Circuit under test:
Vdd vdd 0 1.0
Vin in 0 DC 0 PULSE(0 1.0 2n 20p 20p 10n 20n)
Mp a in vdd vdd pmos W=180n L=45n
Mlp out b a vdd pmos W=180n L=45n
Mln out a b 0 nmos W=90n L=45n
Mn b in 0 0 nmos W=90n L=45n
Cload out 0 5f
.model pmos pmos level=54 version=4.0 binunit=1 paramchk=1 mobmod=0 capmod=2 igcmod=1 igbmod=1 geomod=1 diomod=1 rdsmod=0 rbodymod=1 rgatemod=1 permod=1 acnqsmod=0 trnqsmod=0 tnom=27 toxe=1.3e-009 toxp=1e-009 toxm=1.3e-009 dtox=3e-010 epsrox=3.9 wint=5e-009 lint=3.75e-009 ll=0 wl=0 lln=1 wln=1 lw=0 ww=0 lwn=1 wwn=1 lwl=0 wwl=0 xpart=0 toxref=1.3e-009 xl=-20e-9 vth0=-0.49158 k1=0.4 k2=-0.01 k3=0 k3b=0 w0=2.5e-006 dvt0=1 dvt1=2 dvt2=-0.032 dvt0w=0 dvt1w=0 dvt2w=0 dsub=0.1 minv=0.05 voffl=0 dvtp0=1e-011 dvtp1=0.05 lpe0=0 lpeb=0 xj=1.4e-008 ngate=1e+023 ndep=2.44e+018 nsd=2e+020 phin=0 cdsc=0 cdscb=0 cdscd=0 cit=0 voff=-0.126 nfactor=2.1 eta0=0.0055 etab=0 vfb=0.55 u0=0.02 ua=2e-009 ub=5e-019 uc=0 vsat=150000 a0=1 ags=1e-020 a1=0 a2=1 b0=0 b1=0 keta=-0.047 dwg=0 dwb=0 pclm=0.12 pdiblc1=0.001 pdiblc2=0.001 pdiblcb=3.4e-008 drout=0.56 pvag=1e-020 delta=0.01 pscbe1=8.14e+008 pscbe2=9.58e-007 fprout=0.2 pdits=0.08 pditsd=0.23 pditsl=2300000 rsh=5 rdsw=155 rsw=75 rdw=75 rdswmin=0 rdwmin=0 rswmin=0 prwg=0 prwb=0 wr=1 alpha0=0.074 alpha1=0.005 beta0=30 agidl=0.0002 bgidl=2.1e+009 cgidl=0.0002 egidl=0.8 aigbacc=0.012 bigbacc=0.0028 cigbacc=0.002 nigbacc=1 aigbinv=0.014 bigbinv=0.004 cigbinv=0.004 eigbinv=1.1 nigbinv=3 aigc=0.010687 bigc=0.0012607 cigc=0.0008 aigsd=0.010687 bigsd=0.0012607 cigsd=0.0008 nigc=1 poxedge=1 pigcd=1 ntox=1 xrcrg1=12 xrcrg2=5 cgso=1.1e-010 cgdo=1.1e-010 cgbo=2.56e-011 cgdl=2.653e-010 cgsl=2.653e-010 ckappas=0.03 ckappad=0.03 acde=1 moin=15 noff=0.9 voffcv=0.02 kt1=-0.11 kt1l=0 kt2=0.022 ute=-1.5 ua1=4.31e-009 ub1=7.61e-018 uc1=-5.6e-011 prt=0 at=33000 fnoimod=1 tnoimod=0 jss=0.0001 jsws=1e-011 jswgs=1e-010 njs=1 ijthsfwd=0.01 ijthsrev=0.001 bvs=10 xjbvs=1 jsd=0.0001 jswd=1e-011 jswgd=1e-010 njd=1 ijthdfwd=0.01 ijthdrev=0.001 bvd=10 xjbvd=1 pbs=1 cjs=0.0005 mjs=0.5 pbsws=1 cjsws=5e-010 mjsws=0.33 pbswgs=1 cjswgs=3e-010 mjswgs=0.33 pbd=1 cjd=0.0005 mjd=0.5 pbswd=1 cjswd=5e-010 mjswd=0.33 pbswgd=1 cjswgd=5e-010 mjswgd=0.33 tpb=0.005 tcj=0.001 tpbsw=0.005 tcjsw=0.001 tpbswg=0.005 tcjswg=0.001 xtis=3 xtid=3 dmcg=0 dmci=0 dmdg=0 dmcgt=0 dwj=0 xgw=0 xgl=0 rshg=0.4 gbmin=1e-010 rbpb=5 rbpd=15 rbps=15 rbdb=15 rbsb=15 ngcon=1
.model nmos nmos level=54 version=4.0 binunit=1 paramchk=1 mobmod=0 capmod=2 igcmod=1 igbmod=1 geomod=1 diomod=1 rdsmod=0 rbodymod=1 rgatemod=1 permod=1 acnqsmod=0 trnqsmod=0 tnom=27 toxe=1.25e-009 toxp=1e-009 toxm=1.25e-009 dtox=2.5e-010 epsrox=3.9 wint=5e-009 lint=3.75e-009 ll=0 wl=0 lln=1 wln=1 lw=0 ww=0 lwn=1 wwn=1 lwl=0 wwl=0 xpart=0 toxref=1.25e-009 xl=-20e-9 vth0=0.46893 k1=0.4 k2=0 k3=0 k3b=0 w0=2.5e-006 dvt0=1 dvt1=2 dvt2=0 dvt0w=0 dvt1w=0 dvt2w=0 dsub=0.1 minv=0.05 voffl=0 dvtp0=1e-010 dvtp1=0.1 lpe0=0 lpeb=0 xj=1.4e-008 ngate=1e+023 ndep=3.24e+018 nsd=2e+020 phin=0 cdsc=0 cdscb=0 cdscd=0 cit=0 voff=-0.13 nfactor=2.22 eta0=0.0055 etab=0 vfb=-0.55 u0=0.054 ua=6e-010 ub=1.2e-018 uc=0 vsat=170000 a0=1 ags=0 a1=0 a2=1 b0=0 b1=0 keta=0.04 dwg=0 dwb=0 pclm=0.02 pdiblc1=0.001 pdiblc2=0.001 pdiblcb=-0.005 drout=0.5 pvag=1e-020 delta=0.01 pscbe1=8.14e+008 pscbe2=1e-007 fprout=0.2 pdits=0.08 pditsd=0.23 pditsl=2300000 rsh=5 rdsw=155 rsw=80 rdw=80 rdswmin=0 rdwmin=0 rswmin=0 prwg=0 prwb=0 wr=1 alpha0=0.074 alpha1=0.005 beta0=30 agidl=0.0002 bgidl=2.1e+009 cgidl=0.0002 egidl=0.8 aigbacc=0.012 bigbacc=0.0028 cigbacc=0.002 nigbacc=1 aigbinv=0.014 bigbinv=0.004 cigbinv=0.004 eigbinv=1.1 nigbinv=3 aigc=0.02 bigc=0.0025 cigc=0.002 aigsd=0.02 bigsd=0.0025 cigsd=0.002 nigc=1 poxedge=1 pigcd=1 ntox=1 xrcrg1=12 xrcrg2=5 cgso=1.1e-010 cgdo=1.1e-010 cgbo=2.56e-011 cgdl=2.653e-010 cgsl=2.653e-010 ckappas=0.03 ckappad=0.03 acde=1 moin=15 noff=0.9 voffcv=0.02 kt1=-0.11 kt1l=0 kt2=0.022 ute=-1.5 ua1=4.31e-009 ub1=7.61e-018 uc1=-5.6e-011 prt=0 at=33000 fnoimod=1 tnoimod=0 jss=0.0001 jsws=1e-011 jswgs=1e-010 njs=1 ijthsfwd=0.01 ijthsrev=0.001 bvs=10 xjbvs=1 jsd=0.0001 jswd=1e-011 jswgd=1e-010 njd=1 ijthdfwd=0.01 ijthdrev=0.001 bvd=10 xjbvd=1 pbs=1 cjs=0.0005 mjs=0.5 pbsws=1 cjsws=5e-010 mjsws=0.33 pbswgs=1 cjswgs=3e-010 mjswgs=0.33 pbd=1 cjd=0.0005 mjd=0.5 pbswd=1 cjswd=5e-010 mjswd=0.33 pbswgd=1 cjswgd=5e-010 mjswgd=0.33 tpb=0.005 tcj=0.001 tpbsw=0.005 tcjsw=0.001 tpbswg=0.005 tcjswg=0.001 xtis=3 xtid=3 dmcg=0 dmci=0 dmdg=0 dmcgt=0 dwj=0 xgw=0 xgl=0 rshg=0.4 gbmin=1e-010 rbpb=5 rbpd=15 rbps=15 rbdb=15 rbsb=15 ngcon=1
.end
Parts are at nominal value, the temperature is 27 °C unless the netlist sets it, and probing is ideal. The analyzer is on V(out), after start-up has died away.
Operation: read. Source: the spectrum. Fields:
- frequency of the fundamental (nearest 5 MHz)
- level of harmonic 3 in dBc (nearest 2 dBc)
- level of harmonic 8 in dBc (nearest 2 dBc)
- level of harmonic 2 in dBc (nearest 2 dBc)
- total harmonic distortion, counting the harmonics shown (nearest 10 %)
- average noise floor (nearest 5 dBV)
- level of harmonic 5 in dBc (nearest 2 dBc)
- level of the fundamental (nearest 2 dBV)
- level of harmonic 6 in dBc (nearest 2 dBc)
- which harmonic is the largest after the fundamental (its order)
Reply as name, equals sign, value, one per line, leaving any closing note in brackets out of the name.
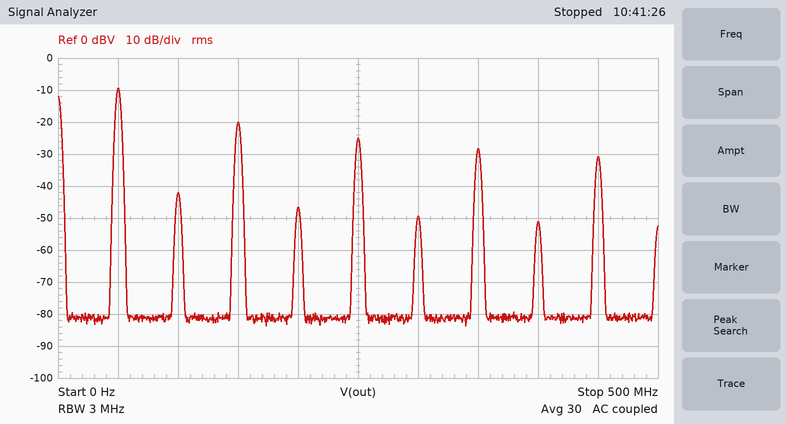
frequency of the fundamental = 50 MHz
level of harmonic 3 in dBc = -10 dBc
level of harmonic 8 in dBc = -42 dBc
level of harmonic 2 in dBc = -32 dBc
total harmonic distortion, counting the harmonics shown = 40 %
average noise floor = -80 dBV
level of harmonic 5 in dBc = -16 dBc
level of the fundamental = -10 dBV
level of harmonic 6 in dBc = -40 dBc
which harmonic is the largest after the fundamental = 3
